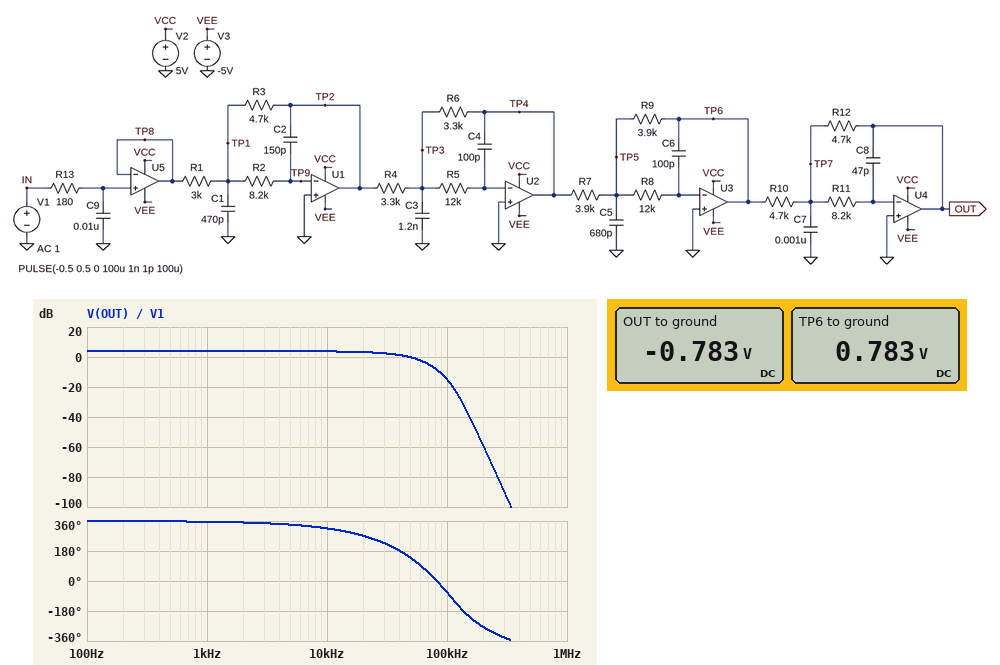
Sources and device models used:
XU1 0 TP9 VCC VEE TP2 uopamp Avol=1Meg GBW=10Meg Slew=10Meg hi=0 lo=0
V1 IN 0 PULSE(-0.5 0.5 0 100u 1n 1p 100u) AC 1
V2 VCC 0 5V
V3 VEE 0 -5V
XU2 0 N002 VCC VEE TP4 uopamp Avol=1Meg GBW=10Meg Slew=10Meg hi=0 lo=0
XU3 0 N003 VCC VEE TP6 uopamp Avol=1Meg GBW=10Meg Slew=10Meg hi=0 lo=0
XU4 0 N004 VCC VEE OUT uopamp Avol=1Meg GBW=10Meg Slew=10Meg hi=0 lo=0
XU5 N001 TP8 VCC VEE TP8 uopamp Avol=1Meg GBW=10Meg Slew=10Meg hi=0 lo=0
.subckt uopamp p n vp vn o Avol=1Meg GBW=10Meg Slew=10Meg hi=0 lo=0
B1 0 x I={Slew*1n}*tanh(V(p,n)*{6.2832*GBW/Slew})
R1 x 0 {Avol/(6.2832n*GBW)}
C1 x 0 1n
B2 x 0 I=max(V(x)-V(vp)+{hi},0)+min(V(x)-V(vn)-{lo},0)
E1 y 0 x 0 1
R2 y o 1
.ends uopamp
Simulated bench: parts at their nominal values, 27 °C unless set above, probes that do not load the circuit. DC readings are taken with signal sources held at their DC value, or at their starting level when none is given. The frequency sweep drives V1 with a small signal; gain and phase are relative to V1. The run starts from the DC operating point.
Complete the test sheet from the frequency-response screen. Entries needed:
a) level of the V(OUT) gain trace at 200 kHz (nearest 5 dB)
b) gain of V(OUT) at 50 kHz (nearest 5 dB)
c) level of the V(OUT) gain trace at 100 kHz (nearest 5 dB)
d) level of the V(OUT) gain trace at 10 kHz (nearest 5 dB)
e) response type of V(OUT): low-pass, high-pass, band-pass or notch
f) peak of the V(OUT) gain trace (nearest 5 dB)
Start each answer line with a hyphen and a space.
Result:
- -60 dB
- 0 dB
- -15 dB
- 5 dB
- low-pass
- 5 dB
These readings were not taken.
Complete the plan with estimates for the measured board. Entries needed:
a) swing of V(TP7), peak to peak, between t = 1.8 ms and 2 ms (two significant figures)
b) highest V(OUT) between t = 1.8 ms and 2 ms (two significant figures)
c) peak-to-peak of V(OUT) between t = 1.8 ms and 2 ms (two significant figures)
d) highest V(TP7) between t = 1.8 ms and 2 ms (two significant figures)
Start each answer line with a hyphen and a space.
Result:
- 79 mV
- 660 mV
- 1.3 V
- 71 mV
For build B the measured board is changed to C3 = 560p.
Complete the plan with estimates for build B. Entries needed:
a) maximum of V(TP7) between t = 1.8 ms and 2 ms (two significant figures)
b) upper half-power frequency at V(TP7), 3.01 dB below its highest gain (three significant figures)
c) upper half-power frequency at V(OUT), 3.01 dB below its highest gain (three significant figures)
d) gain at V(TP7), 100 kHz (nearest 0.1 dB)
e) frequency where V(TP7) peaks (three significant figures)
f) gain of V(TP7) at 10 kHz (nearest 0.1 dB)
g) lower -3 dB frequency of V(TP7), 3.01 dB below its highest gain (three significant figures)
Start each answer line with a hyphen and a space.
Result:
- 67 mV
- 82.4 kHz
- 36.5 kHz
- -25.9 dB
- 47.5 kHz
- -28.3 dB
- 21.9 kHz
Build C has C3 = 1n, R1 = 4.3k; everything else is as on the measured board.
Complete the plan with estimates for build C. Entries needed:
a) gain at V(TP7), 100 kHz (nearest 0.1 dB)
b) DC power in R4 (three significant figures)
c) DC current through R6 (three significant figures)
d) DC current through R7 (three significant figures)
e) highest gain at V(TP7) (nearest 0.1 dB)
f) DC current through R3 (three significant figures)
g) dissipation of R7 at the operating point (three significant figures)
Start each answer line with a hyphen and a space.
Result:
- -28.0 dB
- 90.5 µW
- 166 µA
- 140 µA
- -20.7 dB
- 116 µA
- 76.6 µW
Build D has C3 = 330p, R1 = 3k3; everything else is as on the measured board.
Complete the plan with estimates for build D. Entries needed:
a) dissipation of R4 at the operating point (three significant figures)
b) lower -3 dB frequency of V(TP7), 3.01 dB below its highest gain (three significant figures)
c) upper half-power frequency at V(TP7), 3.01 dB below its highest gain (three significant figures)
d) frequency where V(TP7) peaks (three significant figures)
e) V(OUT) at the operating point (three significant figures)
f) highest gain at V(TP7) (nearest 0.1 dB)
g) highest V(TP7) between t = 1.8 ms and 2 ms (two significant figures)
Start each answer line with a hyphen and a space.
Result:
- 154 µW
- 21.5 kHz
- 82.8 kHz
- 46.9 kHz
- -712 mV
- -20.4 dB
- 60 mV
